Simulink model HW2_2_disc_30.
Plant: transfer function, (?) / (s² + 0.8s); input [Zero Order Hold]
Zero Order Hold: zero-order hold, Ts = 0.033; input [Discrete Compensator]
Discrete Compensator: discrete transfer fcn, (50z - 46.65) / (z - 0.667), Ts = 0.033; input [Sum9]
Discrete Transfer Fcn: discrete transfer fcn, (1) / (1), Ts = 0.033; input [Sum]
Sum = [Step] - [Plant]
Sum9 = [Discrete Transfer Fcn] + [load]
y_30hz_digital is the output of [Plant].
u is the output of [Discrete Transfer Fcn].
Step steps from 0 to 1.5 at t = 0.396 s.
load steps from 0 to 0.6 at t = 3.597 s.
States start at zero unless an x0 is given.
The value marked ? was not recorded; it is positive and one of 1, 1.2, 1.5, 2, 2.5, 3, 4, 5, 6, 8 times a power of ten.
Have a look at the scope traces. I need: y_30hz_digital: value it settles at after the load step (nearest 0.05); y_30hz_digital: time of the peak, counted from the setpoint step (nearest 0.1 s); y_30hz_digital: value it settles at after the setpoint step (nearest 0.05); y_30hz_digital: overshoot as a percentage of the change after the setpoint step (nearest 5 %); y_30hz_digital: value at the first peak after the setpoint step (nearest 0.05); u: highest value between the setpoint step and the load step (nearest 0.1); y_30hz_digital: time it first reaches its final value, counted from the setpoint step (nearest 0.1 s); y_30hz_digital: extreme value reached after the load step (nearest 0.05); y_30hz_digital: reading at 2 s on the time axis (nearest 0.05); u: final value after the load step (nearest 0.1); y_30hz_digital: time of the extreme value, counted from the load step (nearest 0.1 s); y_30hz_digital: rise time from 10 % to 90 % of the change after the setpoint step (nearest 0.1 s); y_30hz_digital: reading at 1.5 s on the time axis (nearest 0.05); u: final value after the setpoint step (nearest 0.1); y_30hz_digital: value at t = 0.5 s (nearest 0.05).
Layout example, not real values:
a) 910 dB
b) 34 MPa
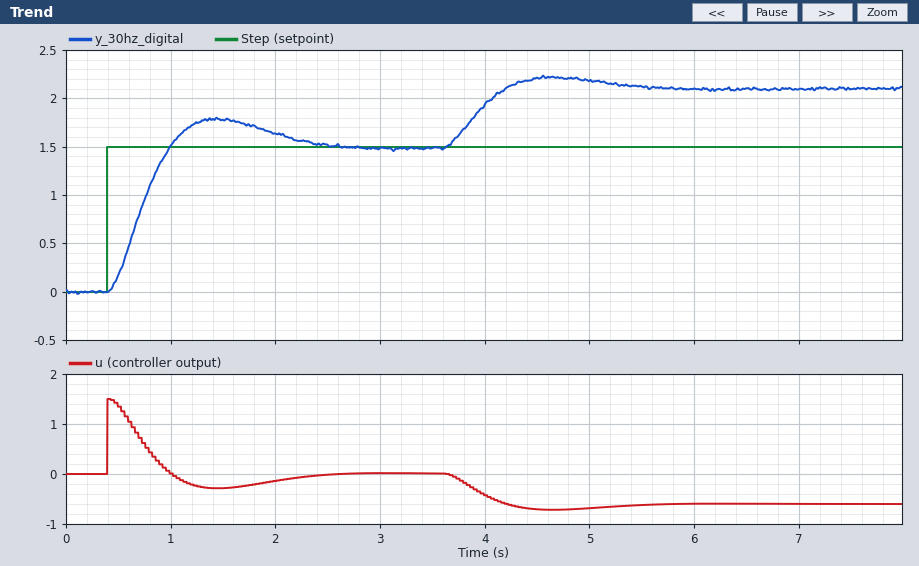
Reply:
a) 2.10
b) 1.0 s
c) 1.50
d) 20 %
e) 1.80
f) 1.5
g) 0.6 s
h) 2.20
i) 1.65
j) -0.6
k) 1.0 s
l) 0.4 s
m) 1.80
n) 0.0
o) 0.15
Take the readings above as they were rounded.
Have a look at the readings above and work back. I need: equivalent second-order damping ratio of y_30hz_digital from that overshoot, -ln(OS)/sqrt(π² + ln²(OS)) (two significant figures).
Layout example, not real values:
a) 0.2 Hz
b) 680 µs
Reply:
a) 0.46
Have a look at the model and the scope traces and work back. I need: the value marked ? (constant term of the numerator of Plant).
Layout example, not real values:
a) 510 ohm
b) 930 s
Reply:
a) 0.5
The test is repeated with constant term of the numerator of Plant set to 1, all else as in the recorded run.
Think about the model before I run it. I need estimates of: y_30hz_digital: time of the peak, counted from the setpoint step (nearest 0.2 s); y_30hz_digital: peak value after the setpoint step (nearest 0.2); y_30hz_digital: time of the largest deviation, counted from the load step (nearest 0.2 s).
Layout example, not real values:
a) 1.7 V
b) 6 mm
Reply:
a) 0.6 s
b) 1.8
c) 0.6 s
